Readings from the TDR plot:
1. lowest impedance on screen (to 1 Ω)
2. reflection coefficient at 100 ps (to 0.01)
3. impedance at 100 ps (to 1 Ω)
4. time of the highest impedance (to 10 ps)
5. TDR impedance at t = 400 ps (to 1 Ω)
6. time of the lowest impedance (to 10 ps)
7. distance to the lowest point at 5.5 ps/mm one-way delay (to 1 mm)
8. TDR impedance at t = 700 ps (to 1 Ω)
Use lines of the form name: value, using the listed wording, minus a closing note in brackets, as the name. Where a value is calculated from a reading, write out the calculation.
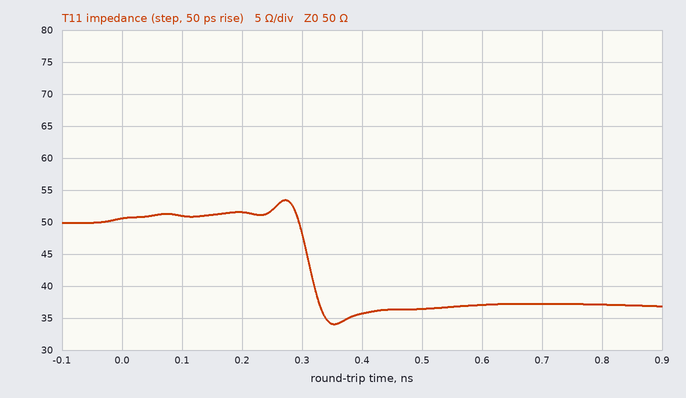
lowest impedance on screen: 34 Ω
reflection coefficient at 100 ps: (51 − 50)/(51 + 50) ≈ +0.01
impedance at 100 ps: 51 Ω
time of the highest impedance: 270 ps
TDR impedance at t = 400 ps: 36 Ω
time of the lowest impedance: 350 ps
distance to the lowest point at 5.5 ps/mm one-way delay: 350 ps / 2 / 5.5 ps/mm ≈ 32 mm
TDR impedance at t = 700 ps: 37 Ω
